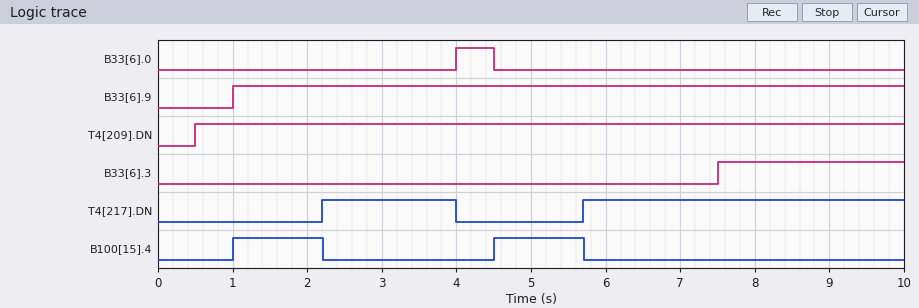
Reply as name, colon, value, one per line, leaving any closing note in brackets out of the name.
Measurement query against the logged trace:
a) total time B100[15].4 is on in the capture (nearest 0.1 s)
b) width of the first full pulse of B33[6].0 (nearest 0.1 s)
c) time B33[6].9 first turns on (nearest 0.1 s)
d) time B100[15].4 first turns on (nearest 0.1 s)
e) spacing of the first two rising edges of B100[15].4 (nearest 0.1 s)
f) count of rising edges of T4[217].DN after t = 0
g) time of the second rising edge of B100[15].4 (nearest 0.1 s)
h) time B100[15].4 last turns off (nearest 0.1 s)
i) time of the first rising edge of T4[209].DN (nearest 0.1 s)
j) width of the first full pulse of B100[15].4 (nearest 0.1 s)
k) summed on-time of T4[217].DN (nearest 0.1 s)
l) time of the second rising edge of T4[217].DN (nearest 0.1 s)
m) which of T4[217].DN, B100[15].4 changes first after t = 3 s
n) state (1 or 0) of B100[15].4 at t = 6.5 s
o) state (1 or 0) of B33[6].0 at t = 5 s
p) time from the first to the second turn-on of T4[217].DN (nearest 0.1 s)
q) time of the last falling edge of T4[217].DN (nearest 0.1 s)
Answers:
total time B100[15].4 is on in the capture: 2.4 s
width of the first full pulse of B33[6].0: 0.5 s
time B33[6].9 first turns on: 1.0 s
time B100[15].4 first turns on: 1.0 s
spacing of the first two rising edges of B100[15].4: 3.5 s
count of rising edges of T4[217].DN after t = 0: 2
time of the second rising edge of B100[15].4: 4.5 s
time B100[15].4 last turns off: 5.7 s
time of the first rising edge of T4[209].DN: 0.5 s
width of the first full pulse of B100[15].4: 1.2 s
summed on-time of T4[217].DN: 6.1 s
time of the second rising edge of T4[217].DN: 5.7 s
which of T4[217].DN, B100[15].4 changes first after t = 3 s: T4[217].DN
state (1 or 0) of B100[15].4 at t = 6.5 s: 0
state (1 or 0) of B33[6].0 at t = 5 s: 0
time from the first to the second turn-on of T4[217].DN: 3.5 s
time of the last falling edge of T4[217].DN: 4.0 s
